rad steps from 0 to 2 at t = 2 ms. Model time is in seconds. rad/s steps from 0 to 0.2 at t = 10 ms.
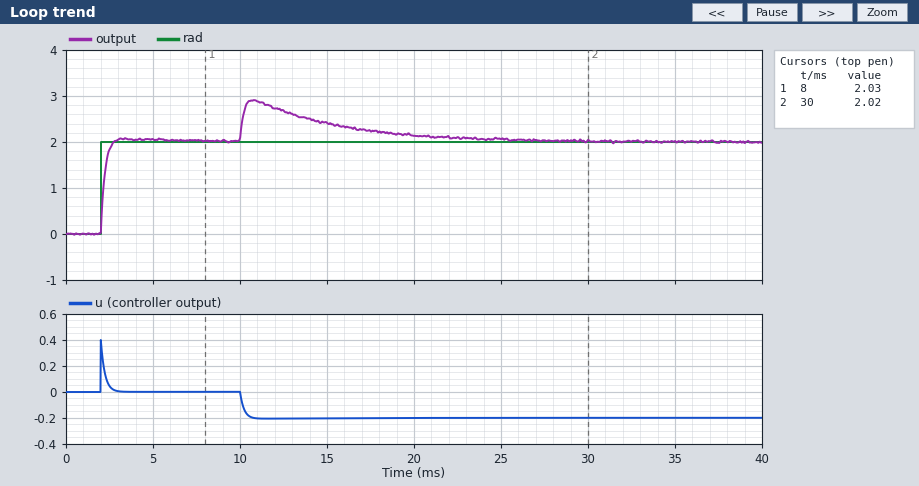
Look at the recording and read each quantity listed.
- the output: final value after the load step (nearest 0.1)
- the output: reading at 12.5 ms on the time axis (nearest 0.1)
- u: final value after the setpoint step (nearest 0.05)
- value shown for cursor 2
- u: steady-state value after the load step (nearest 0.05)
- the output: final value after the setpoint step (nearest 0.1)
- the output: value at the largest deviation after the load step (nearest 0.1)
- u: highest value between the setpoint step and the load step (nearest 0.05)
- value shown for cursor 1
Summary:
2.0
2.7
0.00
2.02
-0.20
2.0
2.9
0.40
2.03
